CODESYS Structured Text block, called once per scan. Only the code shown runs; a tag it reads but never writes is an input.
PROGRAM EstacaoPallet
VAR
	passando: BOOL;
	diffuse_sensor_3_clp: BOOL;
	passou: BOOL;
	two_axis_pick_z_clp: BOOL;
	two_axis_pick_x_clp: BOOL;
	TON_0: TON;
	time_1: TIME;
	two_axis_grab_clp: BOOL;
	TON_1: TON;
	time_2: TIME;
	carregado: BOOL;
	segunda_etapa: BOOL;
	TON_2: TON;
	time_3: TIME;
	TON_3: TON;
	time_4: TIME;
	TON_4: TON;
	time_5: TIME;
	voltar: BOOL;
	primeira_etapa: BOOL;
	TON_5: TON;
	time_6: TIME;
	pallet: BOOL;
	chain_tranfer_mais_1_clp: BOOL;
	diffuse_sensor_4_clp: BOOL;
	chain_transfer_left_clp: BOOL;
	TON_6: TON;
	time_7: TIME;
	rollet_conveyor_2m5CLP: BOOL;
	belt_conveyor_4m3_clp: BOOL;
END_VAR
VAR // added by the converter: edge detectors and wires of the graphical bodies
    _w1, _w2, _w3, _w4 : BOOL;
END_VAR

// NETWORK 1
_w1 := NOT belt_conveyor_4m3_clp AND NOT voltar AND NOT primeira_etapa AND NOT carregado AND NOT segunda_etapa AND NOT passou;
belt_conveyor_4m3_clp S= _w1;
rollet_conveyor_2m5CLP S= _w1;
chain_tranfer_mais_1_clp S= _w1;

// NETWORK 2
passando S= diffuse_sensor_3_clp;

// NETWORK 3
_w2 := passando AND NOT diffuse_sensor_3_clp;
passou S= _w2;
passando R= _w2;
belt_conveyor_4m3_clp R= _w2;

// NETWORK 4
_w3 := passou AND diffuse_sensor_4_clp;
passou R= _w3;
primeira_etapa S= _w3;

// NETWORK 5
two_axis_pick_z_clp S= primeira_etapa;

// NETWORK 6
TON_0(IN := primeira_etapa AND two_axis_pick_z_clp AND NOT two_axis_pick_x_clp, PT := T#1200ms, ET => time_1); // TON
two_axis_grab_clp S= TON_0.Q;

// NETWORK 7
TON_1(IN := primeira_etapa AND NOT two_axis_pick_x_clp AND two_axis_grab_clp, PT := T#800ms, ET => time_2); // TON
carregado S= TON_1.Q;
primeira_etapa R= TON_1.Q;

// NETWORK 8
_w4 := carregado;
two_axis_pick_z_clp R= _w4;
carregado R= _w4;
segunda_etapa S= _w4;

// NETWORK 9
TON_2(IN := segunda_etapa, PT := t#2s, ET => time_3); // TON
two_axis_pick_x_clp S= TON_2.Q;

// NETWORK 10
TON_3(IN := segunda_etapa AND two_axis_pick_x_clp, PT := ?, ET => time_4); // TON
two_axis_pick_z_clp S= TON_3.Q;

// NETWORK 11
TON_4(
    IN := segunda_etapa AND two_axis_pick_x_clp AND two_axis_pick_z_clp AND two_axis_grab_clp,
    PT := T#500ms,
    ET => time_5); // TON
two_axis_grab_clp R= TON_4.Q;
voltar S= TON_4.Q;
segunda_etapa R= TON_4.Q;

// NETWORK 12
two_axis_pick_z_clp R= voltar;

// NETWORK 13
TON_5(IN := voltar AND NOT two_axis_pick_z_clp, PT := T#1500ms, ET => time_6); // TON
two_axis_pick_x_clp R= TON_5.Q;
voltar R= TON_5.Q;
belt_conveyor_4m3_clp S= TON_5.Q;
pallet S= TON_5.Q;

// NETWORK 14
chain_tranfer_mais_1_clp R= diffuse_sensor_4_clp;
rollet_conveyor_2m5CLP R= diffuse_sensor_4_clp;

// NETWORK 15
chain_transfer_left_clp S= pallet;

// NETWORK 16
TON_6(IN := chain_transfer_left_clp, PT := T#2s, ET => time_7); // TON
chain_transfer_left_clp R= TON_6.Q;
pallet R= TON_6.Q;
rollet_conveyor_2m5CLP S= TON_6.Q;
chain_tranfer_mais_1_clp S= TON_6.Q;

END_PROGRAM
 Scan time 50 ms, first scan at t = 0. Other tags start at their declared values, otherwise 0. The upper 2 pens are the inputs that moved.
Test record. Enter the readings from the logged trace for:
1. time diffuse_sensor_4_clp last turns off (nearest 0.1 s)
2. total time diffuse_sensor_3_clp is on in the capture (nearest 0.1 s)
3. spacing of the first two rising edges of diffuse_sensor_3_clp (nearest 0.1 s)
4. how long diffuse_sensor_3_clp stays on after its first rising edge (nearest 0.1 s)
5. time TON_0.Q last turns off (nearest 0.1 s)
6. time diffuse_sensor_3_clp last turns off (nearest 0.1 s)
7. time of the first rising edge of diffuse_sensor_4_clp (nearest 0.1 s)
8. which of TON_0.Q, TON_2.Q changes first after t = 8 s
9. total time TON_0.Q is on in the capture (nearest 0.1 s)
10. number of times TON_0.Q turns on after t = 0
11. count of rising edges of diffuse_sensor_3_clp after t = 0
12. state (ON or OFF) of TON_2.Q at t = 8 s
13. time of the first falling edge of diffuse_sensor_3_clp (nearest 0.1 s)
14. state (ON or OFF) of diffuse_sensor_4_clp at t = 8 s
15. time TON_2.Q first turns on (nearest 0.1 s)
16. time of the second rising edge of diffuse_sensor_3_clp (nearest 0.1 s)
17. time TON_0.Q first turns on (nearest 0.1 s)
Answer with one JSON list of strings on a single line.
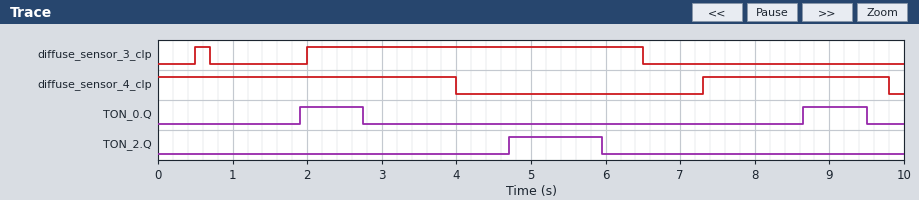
["9.8 s", "4.7 s", "1.5 s", "0.2 s", "9.5 s", "6.5 s", "7.3 s", "TON_0.Q", "1.7 s", "2", "2", "OFF", "0.7 s", "ON", "4.7 s", "2.0 s", "1.9 s"]
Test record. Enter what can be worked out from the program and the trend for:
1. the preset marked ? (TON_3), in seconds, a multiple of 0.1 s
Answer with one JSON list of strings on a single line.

["0.7 s"]
